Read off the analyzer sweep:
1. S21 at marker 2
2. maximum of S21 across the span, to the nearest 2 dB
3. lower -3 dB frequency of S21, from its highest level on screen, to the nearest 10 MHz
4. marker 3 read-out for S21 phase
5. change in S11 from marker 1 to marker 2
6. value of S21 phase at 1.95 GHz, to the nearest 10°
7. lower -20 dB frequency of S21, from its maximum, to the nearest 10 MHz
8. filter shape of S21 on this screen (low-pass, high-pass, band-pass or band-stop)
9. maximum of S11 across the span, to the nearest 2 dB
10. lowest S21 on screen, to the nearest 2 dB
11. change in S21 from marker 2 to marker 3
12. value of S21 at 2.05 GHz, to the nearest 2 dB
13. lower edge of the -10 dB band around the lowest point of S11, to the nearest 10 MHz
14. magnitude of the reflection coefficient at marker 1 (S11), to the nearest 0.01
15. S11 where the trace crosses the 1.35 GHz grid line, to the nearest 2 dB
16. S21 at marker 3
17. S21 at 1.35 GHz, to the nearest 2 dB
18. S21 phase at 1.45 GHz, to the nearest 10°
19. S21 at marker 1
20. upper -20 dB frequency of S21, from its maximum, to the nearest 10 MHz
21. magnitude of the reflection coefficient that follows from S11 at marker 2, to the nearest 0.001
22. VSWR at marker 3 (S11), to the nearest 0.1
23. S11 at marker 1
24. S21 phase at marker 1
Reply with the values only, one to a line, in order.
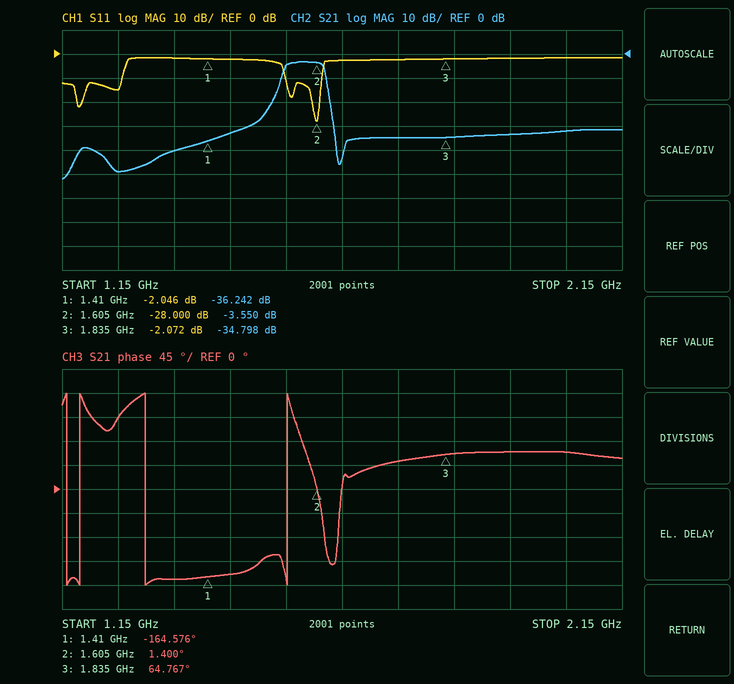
-3.550 dB
-4 dB
1.55 GHz
64.767°
-25.954 dB
70°
1.52 GHz
band-pass
-2 dB
-52 dB
-31.248 dB
-32 dB
1.55 GHz
0.79
-2 dB
-34.798 dB
-40 dB
-160°
-36.242 dB
1.63 GHz
0.040
8.4
-2.046 dB
-164.576°
